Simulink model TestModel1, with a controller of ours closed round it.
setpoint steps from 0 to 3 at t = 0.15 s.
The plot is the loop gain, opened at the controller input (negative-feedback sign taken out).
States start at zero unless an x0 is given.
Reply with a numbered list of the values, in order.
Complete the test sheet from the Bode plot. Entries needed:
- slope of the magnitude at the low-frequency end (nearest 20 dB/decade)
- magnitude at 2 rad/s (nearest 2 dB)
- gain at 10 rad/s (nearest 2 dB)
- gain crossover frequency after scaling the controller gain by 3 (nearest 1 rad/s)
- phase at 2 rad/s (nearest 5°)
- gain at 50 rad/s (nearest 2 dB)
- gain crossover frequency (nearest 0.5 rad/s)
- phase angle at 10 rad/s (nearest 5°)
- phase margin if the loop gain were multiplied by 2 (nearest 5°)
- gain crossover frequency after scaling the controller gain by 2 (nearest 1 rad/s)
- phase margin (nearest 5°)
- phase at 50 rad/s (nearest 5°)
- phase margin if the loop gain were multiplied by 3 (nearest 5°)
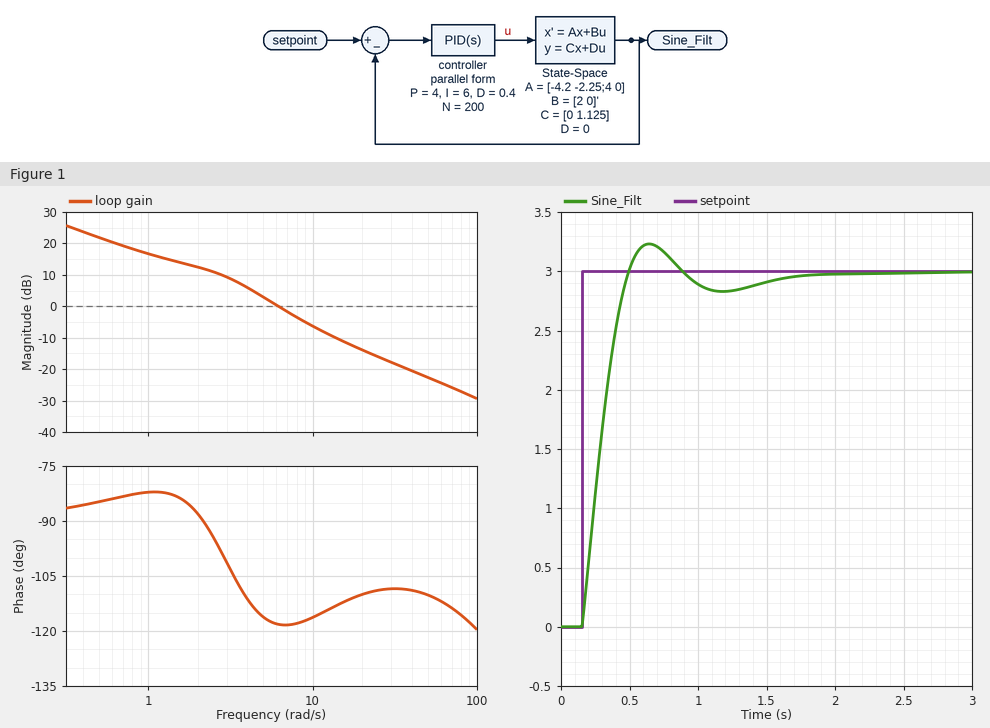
1. -20 dB/decade
2. 12 dB
3. -6 dB
4. 13 rad/s
5. -90°
6. -22 dB
7. 6.0 rad/s
8. -115°
9. 65°
10. 10 rad/s
11. 60°
12. -110°
13. 65°
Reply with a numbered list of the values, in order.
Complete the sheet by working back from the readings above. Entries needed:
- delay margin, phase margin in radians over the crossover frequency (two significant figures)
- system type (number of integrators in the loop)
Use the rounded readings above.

1. 0.17 s
2. 1
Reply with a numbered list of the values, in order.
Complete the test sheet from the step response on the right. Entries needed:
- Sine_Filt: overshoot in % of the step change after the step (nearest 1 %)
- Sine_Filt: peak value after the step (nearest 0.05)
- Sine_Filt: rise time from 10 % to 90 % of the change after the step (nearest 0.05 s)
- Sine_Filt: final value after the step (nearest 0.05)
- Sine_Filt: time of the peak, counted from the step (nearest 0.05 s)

1. 8 %
2. 3.25
3. 0.25 s
4. 3.00
5. 0.50 s
